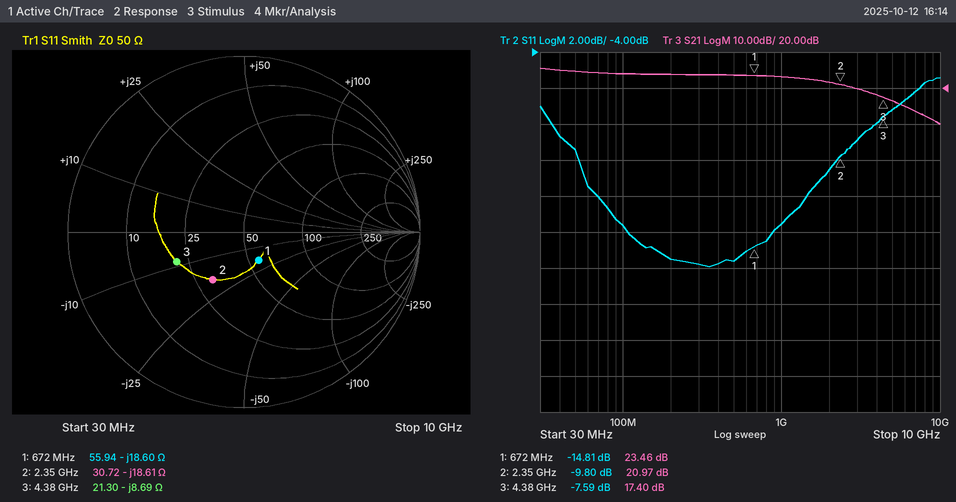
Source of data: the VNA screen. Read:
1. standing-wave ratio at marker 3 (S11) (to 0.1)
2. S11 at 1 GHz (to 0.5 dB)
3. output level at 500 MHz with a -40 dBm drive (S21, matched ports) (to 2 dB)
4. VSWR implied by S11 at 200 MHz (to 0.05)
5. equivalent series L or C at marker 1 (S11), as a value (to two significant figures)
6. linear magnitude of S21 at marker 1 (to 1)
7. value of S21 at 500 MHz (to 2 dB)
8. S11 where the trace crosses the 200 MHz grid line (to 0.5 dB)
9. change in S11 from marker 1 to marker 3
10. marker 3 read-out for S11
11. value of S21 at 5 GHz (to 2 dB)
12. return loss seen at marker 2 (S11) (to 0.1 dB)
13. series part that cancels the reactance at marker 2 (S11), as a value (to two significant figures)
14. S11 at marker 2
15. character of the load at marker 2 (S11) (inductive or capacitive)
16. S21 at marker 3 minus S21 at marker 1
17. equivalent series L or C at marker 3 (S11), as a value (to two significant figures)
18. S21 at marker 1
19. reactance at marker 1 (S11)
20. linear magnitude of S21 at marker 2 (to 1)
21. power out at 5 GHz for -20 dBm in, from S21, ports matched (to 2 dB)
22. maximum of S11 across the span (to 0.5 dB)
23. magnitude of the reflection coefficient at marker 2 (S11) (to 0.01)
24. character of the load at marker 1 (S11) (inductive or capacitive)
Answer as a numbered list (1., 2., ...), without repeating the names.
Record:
1. 2.4
2. -13.5 dB
3. -16 dBm
4. 1.40
5. 13 pF
6. 15
7. 24 dB
8. -15.5 dB
9. 7.22 dB
10. -7.59 dB
11. 16 dB
12. 9.8 dB
13. 1.3 nH
14. -9.80 dB
15. capacitive
16. -6.06 dB
17. 4.2 pF
18. 23.46 dB
19. -18.60 Ω
20. 11
21. -4 dBm
22. -5.5 dB
23. 0.32
24. capacitive
